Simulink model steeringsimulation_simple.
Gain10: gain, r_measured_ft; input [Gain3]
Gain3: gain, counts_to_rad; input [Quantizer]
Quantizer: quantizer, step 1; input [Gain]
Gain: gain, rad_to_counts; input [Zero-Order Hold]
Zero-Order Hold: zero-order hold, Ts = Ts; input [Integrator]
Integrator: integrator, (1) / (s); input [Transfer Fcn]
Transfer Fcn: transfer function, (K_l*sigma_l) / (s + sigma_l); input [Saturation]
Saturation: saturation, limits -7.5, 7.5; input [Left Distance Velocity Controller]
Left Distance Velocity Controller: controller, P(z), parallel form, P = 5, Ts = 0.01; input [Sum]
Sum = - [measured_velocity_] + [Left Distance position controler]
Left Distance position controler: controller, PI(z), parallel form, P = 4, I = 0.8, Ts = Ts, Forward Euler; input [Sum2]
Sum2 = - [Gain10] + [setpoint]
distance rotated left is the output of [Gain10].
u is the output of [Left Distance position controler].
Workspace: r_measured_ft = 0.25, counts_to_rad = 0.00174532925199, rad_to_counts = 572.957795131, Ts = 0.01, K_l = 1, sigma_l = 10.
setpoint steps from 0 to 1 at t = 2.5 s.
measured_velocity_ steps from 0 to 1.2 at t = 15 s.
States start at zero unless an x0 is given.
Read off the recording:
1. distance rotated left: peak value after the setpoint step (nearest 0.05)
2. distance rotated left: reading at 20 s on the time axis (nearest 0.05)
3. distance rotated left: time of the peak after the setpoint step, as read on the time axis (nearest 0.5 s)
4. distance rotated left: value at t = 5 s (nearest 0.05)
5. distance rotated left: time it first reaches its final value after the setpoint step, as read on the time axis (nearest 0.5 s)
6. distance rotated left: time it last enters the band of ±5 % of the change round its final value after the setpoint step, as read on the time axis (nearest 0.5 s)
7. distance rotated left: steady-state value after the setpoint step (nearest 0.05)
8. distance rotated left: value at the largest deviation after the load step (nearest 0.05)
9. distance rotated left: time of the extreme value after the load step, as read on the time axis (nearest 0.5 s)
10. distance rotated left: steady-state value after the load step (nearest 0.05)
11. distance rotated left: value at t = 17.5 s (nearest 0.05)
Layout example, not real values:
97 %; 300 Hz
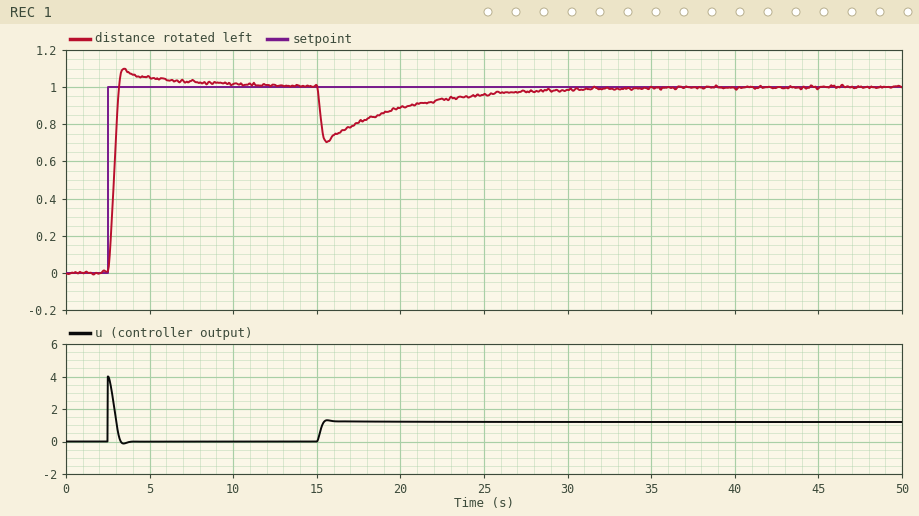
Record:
1.10; 0.90; 3.5 s; 1.05; 3.0 s; 5.0 s; 1.00; 0.70; 15.5 s; 1.00; 0.80
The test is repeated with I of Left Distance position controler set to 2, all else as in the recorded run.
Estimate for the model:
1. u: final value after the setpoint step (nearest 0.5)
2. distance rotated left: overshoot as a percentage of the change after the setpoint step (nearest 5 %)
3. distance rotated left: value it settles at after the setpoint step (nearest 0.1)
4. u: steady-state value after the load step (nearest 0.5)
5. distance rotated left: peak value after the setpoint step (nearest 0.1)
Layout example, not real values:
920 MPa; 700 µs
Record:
0.0; 20 %; 1.0; 1.0; 1.2
